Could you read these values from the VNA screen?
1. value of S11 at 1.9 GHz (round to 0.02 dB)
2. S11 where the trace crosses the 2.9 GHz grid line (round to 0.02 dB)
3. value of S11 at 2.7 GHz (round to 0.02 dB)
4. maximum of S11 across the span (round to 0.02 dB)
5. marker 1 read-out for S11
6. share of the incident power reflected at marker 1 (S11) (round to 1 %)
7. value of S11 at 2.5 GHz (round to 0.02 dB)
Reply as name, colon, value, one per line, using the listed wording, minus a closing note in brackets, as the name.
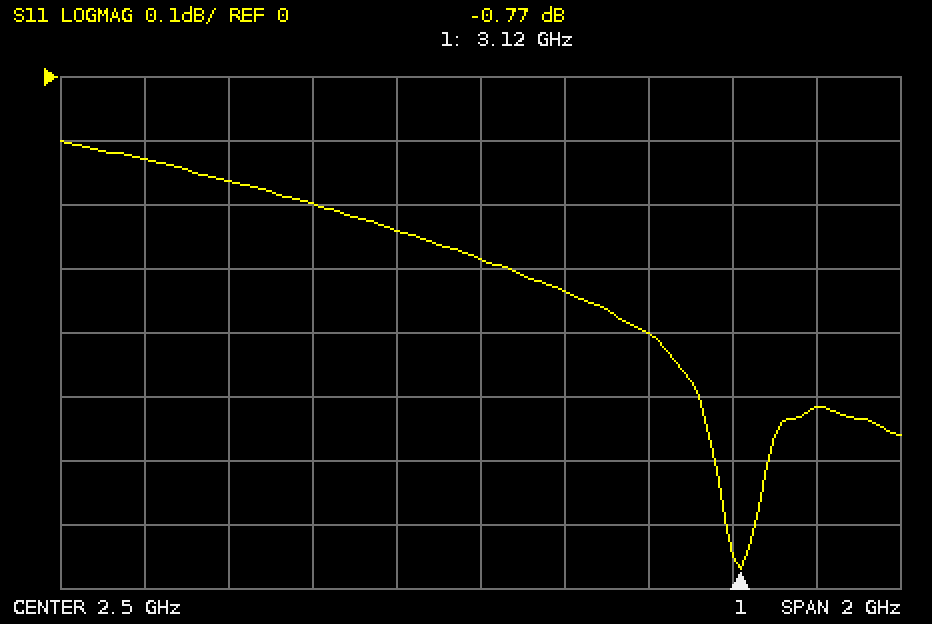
value of S11 at 1.9 GHz: -0.16 dB
S11 where the trace crosses the 2.9 GHz grid line: -0.40 dB
value of S11 at 2.7 GHz: -0.34 dB
maximum of S11 across the span: -0.10 dB
marker 1 read-out for S11: -0.77 dB
share of the incident power reflected at marker 1 (S11): 84 %
value of S11 at 2.5 GHz: -0.28 dB
